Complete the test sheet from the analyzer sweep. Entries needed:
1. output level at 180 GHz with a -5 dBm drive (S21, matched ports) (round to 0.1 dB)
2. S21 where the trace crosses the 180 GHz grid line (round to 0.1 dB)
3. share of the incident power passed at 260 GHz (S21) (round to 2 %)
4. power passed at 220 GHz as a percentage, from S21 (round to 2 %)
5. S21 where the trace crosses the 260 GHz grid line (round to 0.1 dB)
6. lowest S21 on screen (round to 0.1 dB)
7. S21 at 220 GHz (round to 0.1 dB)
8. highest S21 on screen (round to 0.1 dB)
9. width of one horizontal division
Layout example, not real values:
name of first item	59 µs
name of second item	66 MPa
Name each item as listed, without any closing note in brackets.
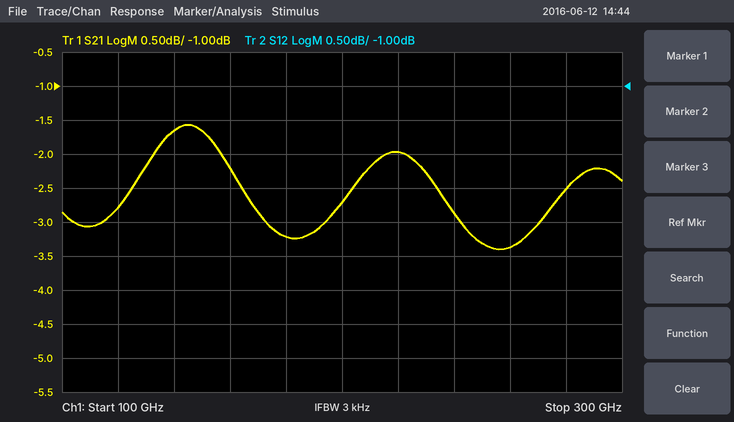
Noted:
output level at 180 GHz with a -5 dBm drive (S21, matched ports)	-8.2 dBm
S21 where the trace crosses the 180 GHz grid line	-3.2 dB
share of the incident power passed at 260 GHz (S21)	46 %
power passed at 220 GHz as a percentage, from S21	64 %
S21 where the trace crosses the 260 GHz grid line	-3.4 dB
lowest S21 on screen	-3.4 dB
S21 at 220 GHz	-2.0 dB
highest S21 on screen	-1.6 dB
width of one horizontal division	20 GHz
